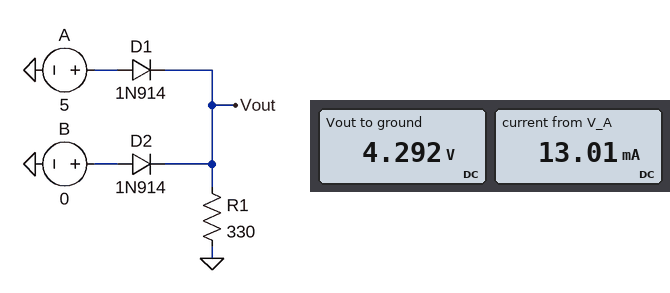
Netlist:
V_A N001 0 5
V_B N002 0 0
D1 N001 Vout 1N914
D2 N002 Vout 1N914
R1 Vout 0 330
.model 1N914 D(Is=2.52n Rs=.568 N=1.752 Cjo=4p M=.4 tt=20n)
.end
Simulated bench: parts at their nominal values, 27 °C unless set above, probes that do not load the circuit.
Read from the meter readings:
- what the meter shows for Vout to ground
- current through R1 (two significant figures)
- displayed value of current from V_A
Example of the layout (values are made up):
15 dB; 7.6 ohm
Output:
4.292 V; 13 mA; 13.01 mA
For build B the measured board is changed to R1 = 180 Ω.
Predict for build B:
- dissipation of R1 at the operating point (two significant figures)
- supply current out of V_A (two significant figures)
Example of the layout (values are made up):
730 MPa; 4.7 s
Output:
100 mW; 24 mA
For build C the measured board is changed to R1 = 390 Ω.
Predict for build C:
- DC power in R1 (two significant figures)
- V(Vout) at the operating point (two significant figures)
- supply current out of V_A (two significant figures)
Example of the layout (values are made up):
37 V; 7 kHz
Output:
47 mW; 4.3 V; 11 mA
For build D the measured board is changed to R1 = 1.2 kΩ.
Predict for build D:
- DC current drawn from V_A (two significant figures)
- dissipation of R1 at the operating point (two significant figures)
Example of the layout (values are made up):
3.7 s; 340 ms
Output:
3.6 mA; 16 mW
